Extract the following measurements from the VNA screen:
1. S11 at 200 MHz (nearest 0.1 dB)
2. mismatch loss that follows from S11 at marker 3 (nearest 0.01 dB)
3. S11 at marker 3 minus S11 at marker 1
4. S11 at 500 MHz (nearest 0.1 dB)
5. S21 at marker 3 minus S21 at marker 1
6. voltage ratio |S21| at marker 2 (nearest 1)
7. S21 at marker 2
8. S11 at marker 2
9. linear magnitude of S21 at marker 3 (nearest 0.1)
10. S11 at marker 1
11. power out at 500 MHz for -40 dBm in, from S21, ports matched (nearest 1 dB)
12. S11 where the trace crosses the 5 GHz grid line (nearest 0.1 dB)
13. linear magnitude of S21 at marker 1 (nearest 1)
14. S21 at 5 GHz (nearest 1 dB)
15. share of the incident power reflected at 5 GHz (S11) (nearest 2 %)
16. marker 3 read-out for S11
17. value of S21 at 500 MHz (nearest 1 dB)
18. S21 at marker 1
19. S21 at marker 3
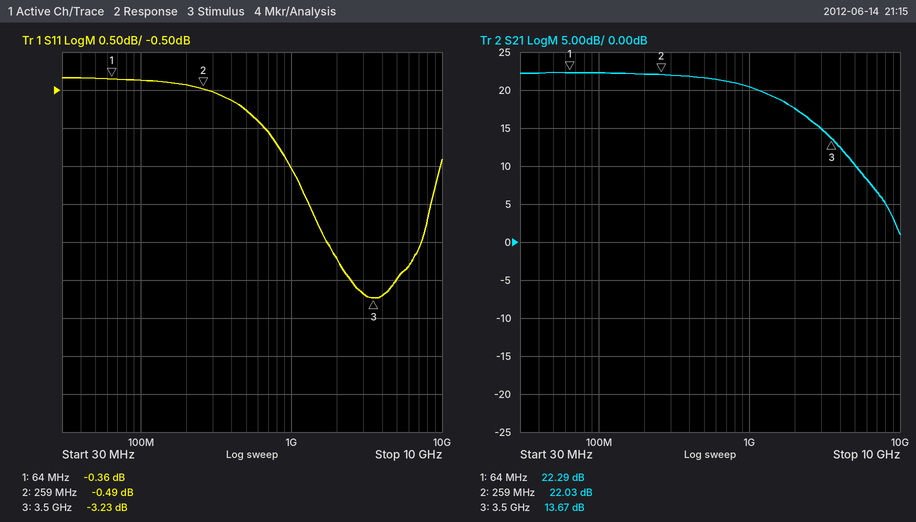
-0.4 dB
2.80 dB
-2.87 dB
-0.8 dB
-8.62 dB
13
22.03 dB
-0.49 dB
4.8
-0.36 dB
-18 dBm
-3.0 dB
13
10 dB
50 %
-3.23 dB
22 dB
22.29 dB
13.67 dB
